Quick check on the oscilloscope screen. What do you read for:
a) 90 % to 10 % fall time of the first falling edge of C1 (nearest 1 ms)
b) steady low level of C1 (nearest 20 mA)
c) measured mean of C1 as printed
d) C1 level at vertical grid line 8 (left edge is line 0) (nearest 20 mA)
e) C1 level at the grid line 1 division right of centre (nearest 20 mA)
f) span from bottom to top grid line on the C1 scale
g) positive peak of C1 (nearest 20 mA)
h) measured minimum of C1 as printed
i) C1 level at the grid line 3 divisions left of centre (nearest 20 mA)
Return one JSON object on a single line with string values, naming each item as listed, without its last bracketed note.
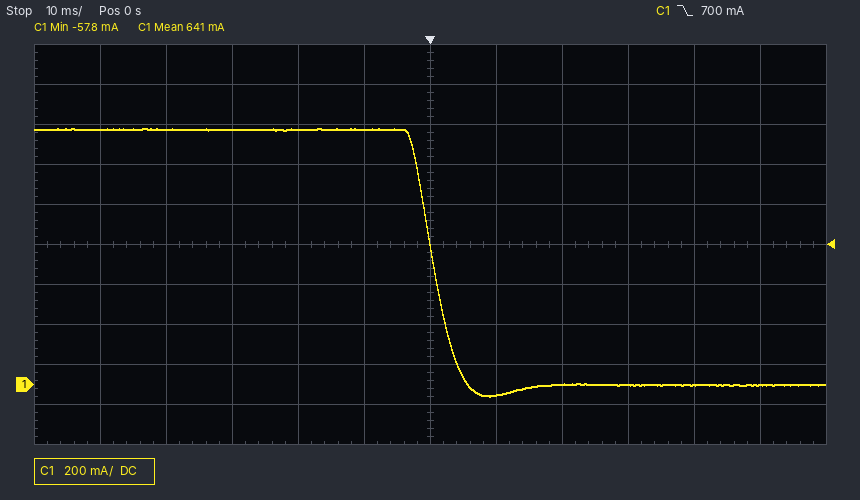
{"90 % to 10 % fall time of the first falling edge of C1": "6 ms", "steady low level of C1": "0 mA", "measured mean of C1 as printed": "641 mA", "C1 level at vertical grid line 8 (left edge is line 0)": "0 mA", "C1 level at the grid line 1 division right of centre": "-60 mA", "span from bottom to top grid line on the C1 scale": "2 A", "positive peak of C1": "1.28 A", "measured minimum of C1 as printed": "-57.8 mA", "C1 level at the grid line 3 divisions left of centre": "1.28 A"}
